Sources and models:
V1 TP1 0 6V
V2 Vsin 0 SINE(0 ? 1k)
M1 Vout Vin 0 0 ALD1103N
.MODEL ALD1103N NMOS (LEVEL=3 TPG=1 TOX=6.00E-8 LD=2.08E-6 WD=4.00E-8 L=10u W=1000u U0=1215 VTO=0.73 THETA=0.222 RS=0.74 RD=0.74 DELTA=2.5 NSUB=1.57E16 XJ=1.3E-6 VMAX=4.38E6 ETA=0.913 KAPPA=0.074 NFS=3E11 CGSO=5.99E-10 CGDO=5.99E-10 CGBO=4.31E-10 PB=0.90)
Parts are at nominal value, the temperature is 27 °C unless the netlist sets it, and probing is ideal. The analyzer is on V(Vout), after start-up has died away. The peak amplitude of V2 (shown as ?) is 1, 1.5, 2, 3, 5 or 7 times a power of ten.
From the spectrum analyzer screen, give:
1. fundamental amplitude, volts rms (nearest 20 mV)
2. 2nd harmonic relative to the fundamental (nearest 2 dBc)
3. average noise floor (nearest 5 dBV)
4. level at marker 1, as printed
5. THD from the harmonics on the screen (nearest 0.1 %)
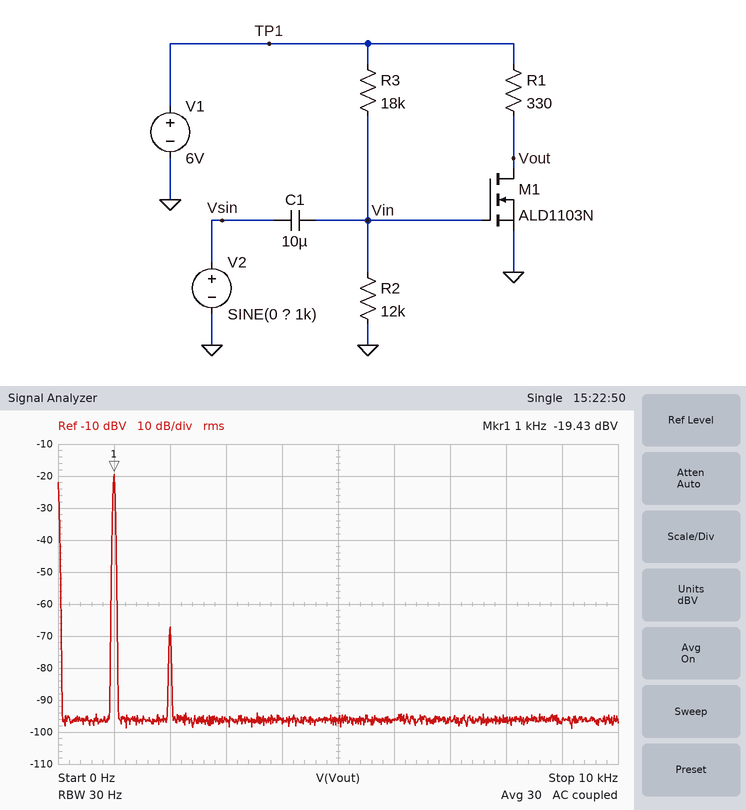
100 mV
-48 dBc
-95 dBV
-19.43 dBV
0.4 %
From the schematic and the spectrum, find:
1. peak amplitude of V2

50 mV
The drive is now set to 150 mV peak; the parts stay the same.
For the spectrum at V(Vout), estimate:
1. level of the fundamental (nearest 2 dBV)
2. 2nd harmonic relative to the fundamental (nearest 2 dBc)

-10 dBV
-38 dBc
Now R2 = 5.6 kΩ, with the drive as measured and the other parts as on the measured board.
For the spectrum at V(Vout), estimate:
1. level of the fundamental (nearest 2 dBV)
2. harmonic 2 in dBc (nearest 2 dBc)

-24 dBV
-38 dBc
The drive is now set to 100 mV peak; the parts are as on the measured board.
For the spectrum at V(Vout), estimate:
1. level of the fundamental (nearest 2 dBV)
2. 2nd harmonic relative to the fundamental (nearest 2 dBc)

-14 dBV
-42 dBc
